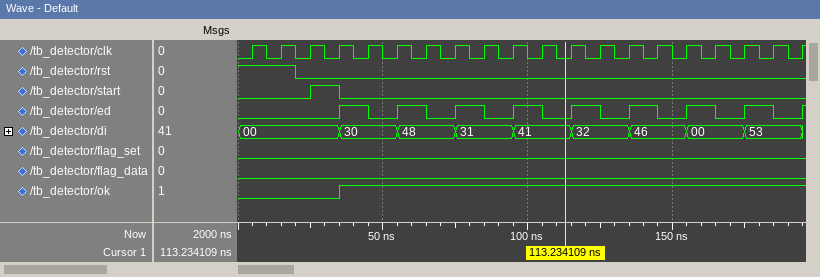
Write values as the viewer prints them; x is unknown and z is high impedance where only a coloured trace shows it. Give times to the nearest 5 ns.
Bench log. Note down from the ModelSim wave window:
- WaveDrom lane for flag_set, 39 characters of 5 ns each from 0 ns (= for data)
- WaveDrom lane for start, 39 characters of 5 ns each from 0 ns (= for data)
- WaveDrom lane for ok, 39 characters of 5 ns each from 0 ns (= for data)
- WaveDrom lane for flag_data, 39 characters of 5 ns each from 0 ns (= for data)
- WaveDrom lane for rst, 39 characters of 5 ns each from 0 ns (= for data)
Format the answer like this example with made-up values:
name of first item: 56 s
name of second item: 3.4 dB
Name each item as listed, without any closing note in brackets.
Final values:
WaveDrom lane for flag_set, 39 characters of 5 ns each from 0 ns: {name: 'flag_set', wave: '0......................................'}
WaveDrom lane for start, 39 characters of 5 ns each from 0 ns: {name: 'start', wave: '0....1.0...............................'}
WaveDrom lane for ok, 39 characters of 5 ns each from 0 ns: {name: 'ok', wave: '0......1...............................'}
WaveDrom lane for flag_data, 39 characters of 5 ns each from 0 ns: {name: 'flag_data', wave: '0......................................'}
WaveDrom lane for rst, 39 characters of 5 ns each from 0 ns: {name: 'rst', wave: '1...0..................................'}
